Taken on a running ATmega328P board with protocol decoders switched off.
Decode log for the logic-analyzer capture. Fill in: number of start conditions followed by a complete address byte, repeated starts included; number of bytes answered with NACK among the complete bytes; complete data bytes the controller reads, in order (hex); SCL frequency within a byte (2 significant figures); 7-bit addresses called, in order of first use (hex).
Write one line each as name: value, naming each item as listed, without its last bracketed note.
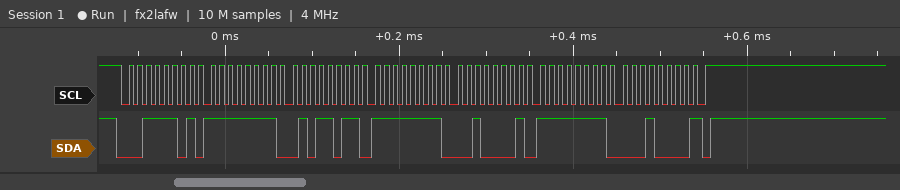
number of start conditions followed by a complete address byte, repeated starts included: 1
number of bytes answered with NACK among the complete bytes: 1
complete data bytes the controller reads, in order: FF 5B FF 21 FF 10
SCL frequency within a byte: 100 kHz
7-bit addresses called, in order of first use: 0x1E
